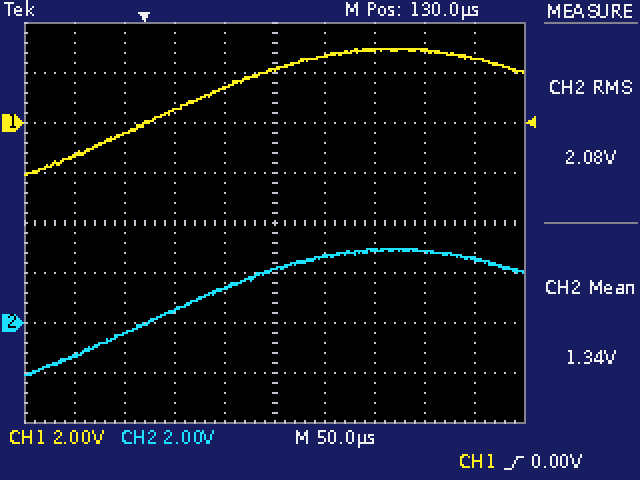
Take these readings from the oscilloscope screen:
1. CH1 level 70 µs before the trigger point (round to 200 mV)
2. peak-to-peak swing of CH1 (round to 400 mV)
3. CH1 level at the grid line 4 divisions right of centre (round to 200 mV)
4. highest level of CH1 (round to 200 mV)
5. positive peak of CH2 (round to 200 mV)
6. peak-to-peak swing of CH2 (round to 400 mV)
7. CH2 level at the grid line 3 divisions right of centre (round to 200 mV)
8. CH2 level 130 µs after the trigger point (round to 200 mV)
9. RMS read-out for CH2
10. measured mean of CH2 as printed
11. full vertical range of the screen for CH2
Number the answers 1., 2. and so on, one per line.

1. -1.4 V
2. 5.2 V
3. 2.6 V
4. 3.0 V
5. 3.0 V
6. 5.2 V
7. 2.8 V
8. 2.2 V
9. 2.08 V
10. 1.34 V
11. 16 V
